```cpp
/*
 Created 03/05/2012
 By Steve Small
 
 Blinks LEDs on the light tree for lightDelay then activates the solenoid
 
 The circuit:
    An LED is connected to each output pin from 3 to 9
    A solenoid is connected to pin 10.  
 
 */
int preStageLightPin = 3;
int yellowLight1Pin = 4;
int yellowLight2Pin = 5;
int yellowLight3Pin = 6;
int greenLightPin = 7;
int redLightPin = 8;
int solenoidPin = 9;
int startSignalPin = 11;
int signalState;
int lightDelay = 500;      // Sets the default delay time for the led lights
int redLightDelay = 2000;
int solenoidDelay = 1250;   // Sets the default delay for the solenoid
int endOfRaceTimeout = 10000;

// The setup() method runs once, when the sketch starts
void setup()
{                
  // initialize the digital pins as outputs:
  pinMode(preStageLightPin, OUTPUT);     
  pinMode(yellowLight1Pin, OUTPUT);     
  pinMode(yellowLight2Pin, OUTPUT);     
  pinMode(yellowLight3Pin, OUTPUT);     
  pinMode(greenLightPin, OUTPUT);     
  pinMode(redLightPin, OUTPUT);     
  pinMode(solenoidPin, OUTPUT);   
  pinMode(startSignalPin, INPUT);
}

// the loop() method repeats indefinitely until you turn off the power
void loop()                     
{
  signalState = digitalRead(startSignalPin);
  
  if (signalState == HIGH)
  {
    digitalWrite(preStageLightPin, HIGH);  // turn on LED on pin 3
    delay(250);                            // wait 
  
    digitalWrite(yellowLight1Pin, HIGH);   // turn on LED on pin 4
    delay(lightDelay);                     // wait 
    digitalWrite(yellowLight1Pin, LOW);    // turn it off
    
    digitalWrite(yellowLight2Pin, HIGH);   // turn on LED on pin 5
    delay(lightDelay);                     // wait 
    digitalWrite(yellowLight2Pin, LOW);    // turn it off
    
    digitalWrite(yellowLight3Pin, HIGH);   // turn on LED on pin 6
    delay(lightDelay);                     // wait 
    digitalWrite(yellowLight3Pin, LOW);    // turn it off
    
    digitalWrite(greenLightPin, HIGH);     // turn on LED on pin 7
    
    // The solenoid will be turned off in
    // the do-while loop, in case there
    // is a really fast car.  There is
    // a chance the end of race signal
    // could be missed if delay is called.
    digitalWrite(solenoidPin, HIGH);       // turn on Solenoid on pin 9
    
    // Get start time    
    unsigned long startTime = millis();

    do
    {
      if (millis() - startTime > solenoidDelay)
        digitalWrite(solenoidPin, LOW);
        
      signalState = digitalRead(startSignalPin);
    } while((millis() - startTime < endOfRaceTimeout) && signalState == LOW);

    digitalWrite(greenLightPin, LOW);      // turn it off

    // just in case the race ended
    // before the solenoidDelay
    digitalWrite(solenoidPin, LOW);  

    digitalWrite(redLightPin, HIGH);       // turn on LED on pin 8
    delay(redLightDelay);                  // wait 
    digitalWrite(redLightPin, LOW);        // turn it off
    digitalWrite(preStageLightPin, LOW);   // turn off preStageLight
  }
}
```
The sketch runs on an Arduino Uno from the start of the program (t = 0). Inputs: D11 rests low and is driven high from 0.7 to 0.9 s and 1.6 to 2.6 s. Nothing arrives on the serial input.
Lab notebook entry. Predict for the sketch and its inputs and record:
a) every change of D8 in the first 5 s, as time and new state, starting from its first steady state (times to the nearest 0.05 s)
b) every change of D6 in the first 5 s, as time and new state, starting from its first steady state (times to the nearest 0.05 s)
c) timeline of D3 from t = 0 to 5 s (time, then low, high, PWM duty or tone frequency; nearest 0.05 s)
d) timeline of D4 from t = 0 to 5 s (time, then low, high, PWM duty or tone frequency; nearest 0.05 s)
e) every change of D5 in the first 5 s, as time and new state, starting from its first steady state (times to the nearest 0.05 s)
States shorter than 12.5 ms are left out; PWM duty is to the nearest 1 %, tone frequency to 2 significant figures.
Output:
0 s low; 2.45 s high; 4.45 s low
0 s low; 1.95 s high; 2.45 s low
0 s low; 0.7 s high; 4.45 s low
0 s low; 0.95 s high; 1.45 s low
0 s low; 1.45 s high; 1.95 s low
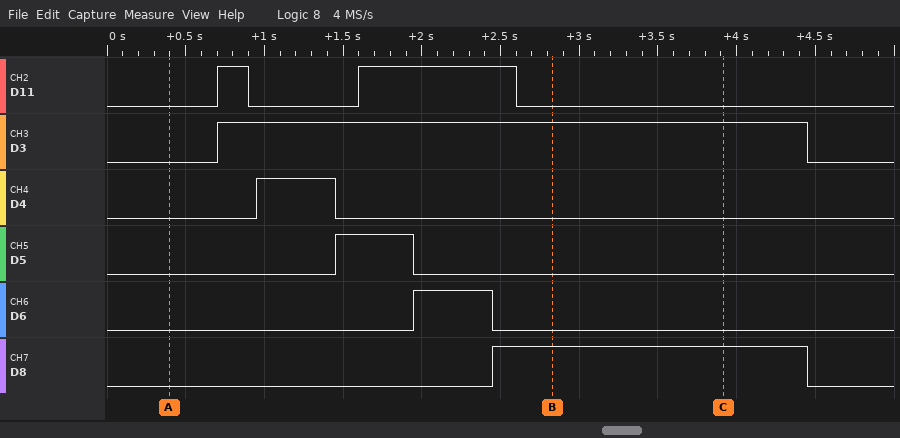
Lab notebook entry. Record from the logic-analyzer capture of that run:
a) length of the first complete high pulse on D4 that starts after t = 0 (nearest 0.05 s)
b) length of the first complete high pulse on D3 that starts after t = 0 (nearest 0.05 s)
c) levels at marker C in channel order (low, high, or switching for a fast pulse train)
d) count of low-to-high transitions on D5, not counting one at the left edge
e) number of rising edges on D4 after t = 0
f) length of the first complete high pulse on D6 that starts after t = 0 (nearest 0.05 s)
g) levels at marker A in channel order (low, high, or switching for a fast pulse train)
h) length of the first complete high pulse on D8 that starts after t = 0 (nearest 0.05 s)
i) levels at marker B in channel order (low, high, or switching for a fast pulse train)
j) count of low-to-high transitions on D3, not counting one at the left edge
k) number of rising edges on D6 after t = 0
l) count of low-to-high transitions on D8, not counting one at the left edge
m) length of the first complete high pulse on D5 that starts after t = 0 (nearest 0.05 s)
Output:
0.50 s
3.75 s
D11 low, D3 high, D4 low, D5 low, D6 low, D8 high
1
1
0.50 s
D11 low, D3 low, D4 low, D5 low, D6 low, D8 low
2.00 s
D11 low, D3 high, D4 low, D5 low, D6 low, D8 high
1
1
1
0.50 s
